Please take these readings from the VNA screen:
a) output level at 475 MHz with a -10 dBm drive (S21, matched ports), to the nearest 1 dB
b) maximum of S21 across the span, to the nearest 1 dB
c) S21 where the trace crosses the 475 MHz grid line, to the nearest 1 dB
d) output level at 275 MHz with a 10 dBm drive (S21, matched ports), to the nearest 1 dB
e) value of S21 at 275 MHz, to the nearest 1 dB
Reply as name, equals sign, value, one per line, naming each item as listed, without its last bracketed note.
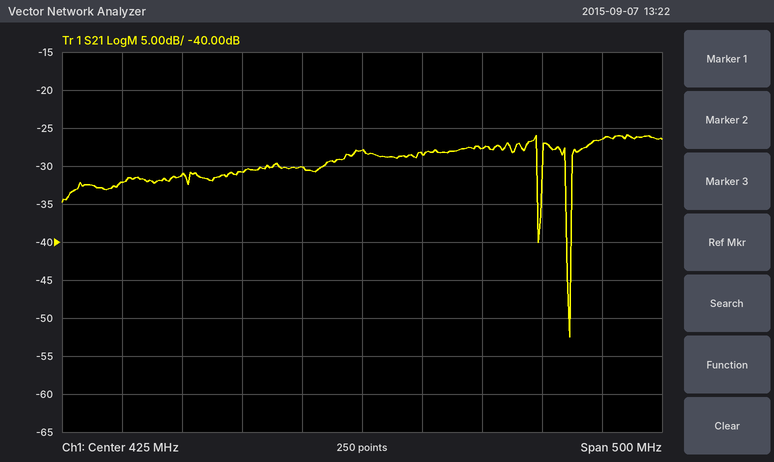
output level at 475 MHz with a -10 dBm drive (S21, matched ports), to the nearest 1 dB = -38 dBm
maximum of S21 across the span, to the nearest 1 dB = -26 dB
S21 where the trace crosses the 475 MHz grid line, to the nearest 1 dB = -28 dB
output level at 275 MHz with a 10 dBm drive (S21, matched ports), to the nearest 1 dB = -21 dBm
value of S21 at 275 MHz, to the nearest 1 dB = -31 dB
